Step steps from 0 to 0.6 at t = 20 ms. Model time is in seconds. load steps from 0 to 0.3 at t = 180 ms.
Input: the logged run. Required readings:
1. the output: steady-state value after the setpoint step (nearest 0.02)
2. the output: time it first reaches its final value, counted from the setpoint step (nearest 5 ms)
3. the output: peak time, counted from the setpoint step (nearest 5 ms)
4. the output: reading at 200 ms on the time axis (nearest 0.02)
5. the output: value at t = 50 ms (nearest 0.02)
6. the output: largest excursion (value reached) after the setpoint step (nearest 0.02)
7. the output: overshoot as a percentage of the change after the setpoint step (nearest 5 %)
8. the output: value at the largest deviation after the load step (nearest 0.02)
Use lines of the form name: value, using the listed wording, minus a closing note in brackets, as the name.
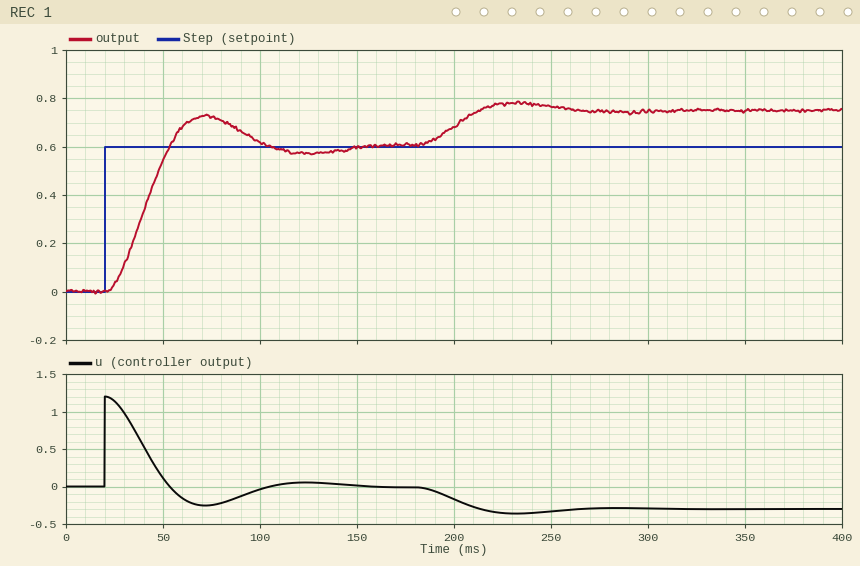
the output: steady-state value after the setpoint step: 0.60
the output: time it first reaches its final value, counted from the setpoint step: 35 ms
the output: peak time, counted from the setpoint step: 50 ms
the output: reading at 200 ms on the time axis: 0.68
the output: value at t = 50 ms: 0.54
the output: largest excursion (value reached) after the setpoint step: 0.72
the output: overshoot as a percentage of the change after the setpoint step: 20 %
the output: value at the largest deviation after the load step: 0.78
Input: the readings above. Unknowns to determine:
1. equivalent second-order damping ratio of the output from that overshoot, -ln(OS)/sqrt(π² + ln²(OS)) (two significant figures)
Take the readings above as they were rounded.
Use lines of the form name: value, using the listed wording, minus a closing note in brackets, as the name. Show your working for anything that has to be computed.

equivalent second-order damping ratio of the output from that overshoot, -ln(OS)/sqrt(π² + ln²(OS)): ln(0.2) = -1.609; 1.609 / sqrt(9.870 + 2.590) = 0.46
